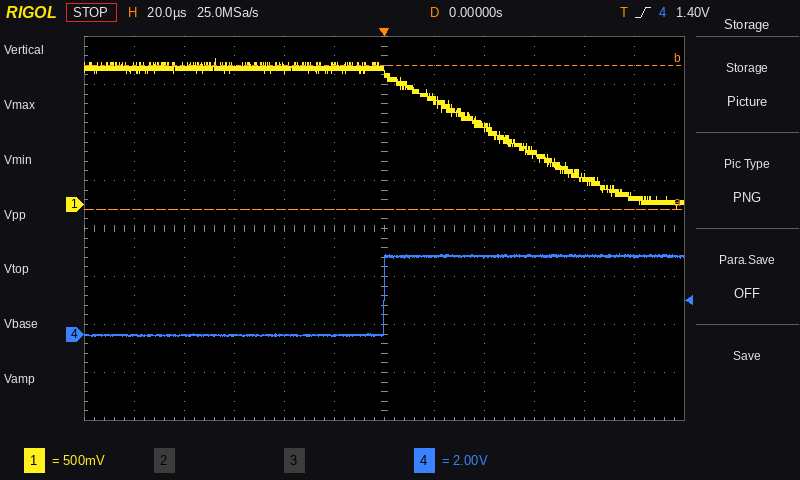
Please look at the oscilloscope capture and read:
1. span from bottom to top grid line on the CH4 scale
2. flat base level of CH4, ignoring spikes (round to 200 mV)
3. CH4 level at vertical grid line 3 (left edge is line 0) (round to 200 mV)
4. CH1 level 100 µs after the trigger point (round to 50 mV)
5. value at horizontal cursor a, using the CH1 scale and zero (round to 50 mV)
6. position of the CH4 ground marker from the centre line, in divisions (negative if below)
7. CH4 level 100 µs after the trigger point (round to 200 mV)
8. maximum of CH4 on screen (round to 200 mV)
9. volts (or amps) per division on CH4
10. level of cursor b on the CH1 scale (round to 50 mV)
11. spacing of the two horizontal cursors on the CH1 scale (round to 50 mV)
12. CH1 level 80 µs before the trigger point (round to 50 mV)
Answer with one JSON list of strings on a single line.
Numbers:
["16 V", "0.0 V", "0.0 V", "50 mV", "-50 mV", "-2.2 div", "3.2 V", "3.4 V", "2 V", "1.45 V", "1.50 V", "1.45 V"]
